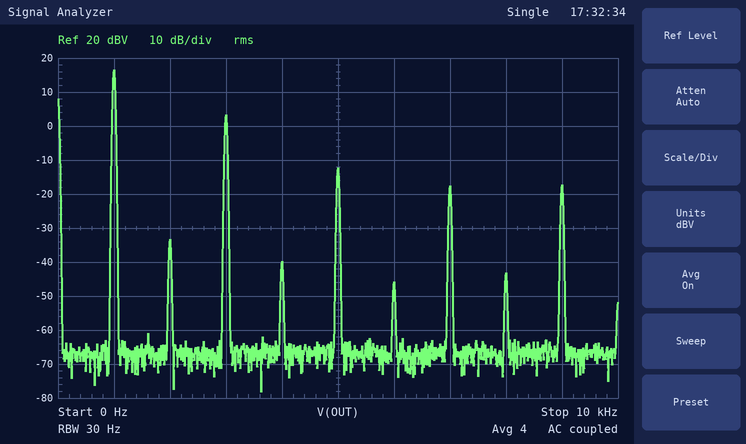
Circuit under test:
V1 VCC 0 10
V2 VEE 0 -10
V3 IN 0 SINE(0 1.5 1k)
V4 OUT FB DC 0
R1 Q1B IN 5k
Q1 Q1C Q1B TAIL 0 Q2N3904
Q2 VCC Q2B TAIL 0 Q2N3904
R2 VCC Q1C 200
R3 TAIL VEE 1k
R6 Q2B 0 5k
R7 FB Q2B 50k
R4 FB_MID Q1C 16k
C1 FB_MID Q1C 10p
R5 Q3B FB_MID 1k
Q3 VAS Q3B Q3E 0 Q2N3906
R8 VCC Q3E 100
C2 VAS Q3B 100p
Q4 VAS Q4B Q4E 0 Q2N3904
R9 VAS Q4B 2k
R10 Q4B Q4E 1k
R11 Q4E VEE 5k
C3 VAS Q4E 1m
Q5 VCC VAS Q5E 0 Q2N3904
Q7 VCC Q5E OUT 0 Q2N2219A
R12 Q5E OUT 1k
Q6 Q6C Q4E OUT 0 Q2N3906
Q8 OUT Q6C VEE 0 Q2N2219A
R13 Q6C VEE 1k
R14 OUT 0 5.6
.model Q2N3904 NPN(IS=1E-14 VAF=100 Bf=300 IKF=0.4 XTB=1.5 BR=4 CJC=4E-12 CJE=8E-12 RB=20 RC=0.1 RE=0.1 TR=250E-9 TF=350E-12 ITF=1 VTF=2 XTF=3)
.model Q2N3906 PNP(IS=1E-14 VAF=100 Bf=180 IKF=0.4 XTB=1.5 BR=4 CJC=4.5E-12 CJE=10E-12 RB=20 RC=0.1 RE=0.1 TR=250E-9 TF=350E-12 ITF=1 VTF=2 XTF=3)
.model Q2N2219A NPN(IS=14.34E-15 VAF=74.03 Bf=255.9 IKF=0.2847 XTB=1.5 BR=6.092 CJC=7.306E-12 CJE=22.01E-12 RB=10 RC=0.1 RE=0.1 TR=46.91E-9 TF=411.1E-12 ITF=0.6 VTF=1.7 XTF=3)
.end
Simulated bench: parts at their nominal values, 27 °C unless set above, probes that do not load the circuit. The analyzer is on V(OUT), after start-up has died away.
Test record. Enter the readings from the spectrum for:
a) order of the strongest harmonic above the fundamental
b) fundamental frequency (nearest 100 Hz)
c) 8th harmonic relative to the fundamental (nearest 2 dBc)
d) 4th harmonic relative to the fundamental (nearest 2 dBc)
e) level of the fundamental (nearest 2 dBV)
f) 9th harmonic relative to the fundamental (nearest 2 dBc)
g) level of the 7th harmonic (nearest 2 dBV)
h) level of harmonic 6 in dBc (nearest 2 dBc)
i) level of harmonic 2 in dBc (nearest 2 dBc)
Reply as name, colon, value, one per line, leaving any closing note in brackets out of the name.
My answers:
order of the strongest harmonic above the fundamental: 3
fundamental frequency: 1.0 kHz
8th harmonic relative to the fundamental: -60 dBc
4th harmonic relative to the fundamental: -56 dBc
level of the fundamental: 16 dBV
9th harmonic relative to the fundamental: -34 dBc
level of the 7th harmonic: -18 dBV
level of harmonic 6 in dBc: -62 dBc
level of harmonic 2 in dBc: -50 dBc
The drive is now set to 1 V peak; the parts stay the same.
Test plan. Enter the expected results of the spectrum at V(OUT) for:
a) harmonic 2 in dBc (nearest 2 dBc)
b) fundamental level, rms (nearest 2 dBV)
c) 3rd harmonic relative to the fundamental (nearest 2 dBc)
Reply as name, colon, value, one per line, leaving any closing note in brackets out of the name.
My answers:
harmonic 2 in dBc: -48 dBc
fundamental level, rms: 16 dBV
3rd harmonic relative to the fundamental: -20 dBc
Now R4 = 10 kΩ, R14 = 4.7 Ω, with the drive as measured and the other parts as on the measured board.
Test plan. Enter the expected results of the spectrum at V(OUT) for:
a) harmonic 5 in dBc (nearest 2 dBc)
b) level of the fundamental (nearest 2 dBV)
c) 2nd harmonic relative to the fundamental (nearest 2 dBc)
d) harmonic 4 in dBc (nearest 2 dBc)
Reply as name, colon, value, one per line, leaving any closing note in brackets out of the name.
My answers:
harmonic 5 in dBc: -26 dBc
level of the fundamental: 16 dBV
2nd harmonic relative to the fundamental: -46 dBc
harmonic 4 in dBc: -52 dBc
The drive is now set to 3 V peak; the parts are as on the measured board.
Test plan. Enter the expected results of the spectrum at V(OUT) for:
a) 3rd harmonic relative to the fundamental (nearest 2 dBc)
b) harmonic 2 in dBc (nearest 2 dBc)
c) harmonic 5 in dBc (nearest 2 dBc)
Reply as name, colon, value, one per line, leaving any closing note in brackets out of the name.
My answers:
3rd harmonic relative to the fundamental: -10 dBc
harmonic 2 in dBc: -58 dBc
harmonic 5 in dBc: -16 dBc
